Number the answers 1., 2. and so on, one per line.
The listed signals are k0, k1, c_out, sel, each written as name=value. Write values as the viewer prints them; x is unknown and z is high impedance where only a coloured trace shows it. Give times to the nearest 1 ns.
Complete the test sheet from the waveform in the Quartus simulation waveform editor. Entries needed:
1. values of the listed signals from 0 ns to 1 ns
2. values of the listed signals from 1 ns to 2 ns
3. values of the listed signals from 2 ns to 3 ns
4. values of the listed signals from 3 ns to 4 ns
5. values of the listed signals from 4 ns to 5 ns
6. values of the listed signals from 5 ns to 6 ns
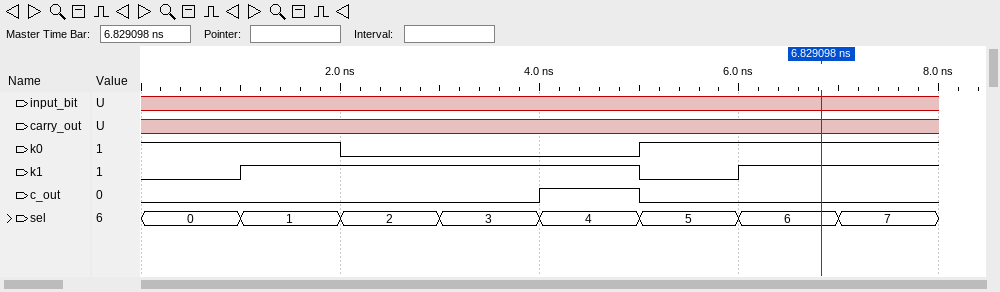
1. k0=1, k1=0, c_out=0, sel=0
2. k0=1, k1=1, c_out=0, sel=1
3. k0=0, k1=1, c_out=0, sel=2
4. k0=0, k1=1, c_out=0, sel=3
5. k0=0, k1=1, c_out=1, sel=4
6. k0=1, k1=0, c_out=0, sel=5
